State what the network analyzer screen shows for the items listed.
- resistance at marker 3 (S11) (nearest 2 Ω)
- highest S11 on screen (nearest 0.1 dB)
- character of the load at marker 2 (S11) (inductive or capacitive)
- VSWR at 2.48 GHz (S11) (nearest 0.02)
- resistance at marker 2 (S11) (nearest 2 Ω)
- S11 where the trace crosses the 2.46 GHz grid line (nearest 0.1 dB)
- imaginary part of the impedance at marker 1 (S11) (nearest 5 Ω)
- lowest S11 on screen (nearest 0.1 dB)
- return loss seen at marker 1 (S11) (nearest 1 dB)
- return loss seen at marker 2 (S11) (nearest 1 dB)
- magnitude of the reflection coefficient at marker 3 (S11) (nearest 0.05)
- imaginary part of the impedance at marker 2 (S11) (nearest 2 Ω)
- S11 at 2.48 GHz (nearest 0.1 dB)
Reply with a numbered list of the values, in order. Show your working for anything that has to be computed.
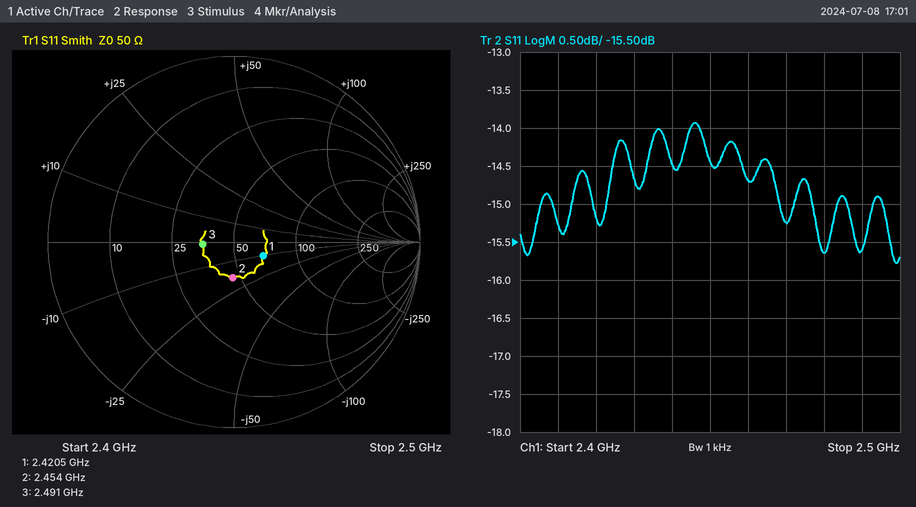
1. 36 Ω
2. -13.9 dB
3. capacitive
4. |Γ| = 10^(-15.6/20) = 0.1660; VSWR = (1 + 0.1660)/(1 − 0.1660) ≈ 1.40
5. 46 Ω
6. -14.7 dB
7. -10 Ω
8. -15.8 dB
9. 15 dB
10. 14 dB
11. 0.15
12. -18 Ω
13. -15.6 dB
